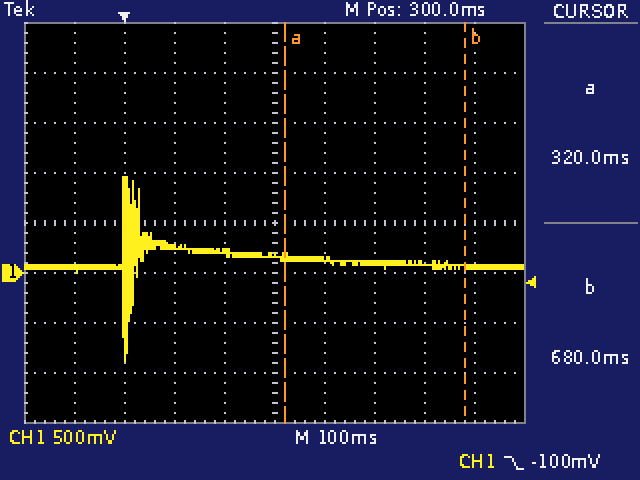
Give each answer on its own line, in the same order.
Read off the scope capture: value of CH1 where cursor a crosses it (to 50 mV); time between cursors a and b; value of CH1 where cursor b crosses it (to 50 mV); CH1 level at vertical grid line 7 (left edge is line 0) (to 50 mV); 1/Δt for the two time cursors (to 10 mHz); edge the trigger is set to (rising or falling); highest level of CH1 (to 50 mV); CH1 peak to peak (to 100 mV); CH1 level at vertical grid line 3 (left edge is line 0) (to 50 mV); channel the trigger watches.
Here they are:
150 mV
360 ms
50 mV
100 mV
2.78 Hz
falling
950 mV
1.80 V
250 mV
CH1
